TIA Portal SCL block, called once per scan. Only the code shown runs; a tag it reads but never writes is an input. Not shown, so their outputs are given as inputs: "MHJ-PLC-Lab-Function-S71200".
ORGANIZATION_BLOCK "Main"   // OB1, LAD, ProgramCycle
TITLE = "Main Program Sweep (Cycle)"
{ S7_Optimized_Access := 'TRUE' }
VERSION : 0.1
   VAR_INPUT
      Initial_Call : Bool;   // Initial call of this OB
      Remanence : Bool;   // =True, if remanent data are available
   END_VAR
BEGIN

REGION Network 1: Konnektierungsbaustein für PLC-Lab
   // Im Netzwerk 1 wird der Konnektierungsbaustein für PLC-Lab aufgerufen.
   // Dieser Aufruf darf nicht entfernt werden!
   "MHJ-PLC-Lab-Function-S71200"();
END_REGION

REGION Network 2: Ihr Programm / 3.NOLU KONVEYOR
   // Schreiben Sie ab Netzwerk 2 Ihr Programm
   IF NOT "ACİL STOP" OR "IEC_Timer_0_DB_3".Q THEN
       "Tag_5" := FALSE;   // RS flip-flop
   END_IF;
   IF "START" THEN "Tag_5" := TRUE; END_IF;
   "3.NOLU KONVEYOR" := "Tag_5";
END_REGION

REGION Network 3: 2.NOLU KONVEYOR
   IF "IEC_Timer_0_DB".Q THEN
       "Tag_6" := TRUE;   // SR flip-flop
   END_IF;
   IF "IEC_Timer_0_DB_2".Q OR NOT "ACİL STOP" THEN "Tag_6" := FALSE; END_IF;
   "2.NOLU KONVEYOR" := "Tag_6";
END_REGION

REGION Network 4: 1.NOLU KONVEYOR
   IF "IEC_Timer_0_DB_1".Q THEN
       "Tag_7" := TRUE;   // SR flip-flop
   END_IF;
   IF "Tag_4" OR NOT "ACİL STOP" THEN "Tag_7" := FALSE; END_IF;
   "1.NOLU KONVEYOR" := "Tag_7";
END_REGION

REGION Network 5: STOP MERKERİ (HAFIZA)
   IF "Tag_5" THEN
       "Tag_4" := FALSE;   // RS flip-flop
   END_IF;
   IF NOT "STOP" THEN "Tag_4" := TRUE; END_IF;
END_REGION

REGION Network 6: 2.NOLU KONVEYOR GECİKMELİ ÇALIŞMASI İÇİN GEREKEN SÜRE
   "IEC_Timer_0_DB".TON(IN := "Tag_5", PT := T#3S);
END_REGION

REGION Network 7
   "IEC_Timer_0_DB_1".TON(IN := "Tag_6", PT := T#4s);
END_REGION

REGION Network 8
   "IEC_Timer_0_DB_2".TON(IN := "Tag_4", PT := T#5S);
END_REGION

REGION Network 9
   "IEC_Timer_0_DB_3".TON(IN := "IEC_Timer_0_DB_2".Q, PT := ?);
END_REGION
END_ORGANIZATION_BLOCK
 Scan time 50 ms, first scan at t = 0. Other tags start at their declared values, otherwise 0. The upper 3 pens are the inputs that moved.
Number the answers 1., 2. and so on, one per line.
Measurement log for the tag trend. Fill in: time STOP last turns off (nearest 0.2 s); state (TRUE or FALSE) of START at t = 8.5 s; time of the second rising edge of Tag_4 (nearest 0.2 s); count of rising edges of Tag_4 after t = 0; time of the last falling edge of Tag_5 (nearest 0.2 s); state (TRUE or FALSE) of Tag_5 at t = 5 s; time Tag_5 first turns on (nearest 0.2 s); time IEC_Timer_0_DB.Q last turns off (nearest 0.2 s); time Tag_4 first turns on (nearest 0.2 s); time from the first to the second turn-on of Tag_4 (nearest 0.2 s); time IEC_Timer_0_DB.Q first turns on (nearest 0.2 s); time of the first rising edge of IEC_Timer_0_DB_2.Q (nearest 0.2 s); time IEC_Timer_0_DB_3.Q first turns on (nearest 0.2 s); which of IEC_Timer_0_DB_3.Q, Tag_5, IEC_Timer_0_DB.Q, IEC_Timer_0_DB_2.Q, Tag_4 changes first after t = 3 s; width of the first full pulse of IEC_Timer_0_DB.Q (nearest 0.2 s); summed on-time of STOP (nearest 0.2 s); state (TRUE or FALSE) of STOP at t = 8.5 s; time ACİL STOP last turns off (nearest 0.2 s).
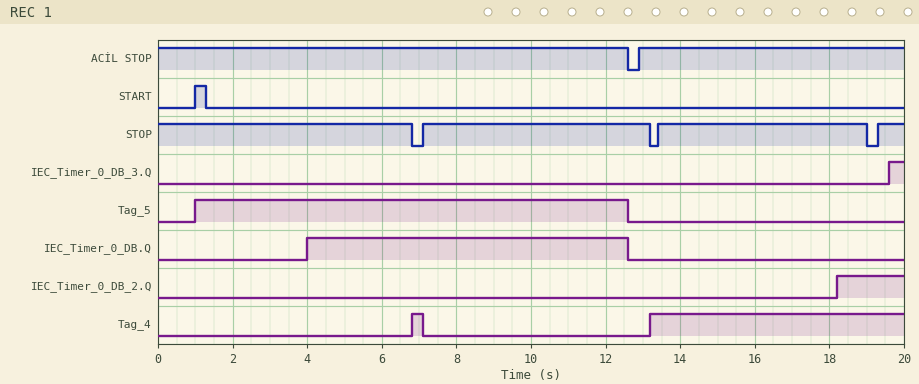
1. 19.0 s
2. FALSE
3. 13.2 s
4. 2
5. 12.6 s
6. TRUE
7. 1.0 s
8. 12.6 s
9. 6.8 s
10. 6.4 s
11. 4.0 s
12. 18.2 s
13. 19.6 s
14. IEC_Timer_0_DB.Q
15. 8.6 s
16. 19.2 s
17. TRUE
18. 12.6 s
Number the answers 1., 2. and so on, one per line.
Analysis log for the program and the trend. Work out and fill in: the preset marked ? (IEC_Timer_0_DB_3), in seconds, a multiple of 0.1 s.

1. 1.4 s
